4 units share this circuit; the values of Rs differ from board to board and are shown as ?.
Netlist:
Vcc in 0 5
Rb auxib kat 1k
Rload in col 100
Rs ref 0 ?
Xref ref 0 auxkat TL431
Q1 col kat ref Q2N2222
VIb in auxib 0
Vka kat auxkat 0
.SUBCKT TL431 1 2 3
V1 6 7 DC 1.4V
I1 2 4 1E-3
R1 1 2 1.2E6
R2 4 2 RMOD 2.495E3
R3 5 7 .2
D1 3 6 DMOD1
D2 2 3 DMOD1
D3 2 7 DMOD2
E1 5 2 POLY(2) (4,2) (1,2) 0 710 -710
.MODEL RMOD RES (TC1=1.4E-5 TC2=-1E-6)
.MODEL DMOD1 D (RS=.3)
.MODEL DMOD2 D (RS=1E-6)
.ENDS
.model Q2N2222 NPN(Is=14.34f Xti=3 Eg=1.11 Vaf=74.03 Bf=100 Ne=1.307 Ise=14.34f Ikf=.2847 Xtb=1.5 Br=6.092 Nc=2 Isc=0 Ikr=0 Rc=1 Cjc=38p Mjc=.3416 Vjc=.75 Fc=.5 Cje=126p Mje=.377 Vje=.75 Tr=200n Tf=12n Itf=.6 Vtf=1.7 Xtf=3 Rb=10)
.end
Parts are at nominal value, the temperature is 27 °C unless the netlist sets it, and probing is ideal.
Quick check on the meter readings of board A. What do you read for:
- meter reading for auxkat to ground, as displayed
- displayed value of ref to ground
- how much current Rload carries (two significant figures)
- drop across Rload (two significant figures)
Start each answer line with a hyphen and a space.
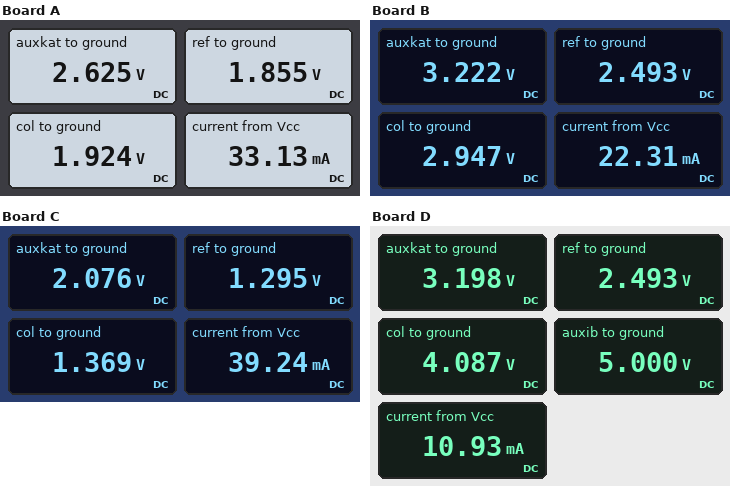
- 2.625 V
- 1.855 V
- 31 mA
- 3.1 V
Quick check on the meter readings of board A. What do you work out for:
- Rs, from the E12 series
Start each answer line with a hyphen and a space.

- 56 Ω
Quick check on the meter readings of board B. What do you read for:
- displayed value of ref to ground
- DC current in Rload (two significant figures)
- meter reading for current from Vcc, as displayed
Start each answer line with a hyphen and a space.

- 2.493 V
- 21 mA
- 22.31 mA
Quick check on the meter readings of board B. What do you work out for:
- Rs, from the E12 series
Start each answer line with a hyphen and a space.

- 120 Ω
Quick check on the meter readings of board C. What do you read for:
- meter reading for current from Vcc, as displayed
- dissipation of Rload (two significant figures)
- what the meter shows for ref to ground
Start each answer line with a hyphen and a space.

- 39.24 mA
- 130 mW
- 1.295 V
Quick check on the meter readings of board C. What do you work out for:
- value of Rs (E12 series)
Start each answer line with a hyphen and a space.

- 33 Ω
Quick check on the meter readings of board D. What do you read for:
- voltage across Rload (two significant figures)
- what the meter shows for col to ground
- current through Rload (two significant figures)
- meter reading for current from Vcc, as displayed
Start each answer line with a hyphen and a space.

- 910 mV
- 4.087 V
- 9.1 mA
- 10.93 mA
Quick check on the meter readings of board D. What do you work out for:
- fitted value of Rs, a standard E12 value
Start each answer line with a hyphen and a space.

- 270 Ω
